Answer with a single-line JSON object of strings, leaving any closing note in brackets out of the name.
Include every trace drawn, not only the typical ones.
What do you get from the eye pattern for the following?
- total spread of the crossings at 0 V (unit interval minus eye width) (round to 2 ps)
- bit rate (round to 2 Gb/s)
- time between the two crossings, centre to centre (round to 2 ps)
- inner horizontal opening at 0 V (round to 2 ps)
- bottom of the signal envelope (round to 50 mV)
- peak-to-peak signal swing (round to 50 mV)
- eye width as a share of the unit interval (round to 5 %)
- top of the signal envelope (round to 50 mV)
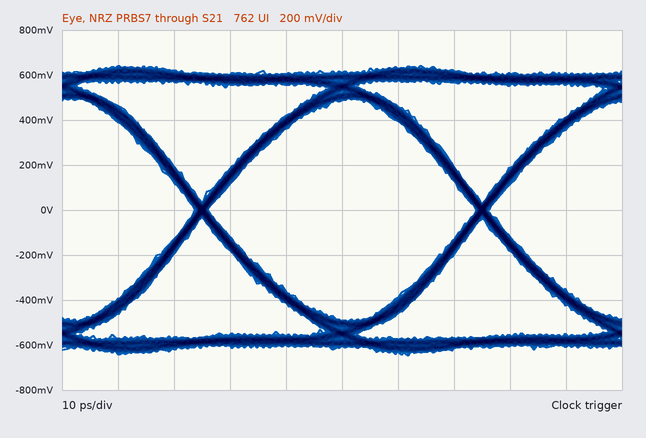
{"total spread of the crossings at 0 V (unit interval minus eye width)": "2 ps", "bit rate": "20 Gb/s", "time between the two crossings, centre to centre": "50 ps", "inner horizontal opening at 0 V": "48 ps", "bottom of the signal envelope": "-650 mV", "peak-to-peak signal swing": "1.30 V", "eye width as a share of the unit interval": "95 %", "top of the signal envelope": "650 mV"}
